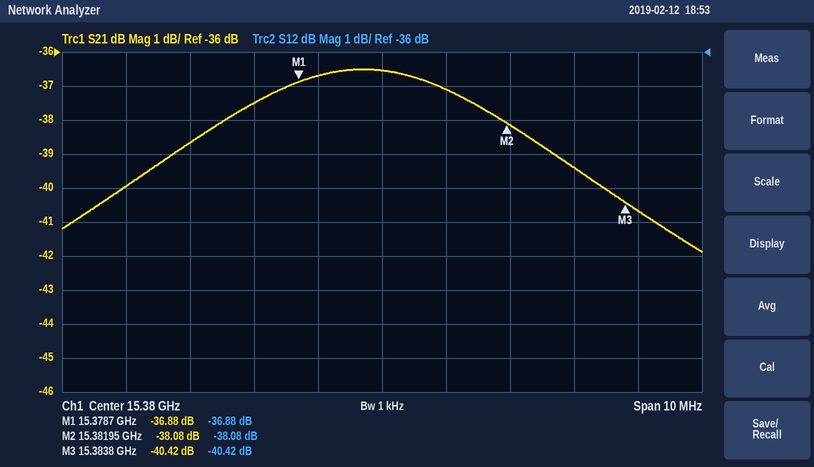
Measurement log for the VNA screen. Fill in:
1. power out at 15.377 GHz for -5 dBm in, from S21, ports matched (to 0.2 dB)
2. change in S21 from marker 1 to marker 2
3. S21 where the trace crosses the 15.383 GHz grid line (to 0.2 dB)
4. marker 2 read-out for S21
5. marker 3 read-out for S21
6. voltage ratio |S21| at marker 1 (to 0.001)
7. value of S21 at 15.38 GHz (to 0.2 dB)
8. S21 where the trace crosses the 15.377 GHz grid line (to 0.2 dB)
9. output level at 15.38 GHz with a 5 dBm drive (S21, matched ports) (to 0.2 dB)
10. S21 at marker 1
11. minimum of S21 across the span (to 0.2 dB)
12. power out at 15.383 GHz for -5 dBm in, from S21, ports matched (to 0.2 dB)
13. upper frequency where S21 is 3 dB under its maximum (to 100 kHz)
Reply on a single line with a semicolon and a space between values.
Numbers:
-43.6 dBm; -1.20 dB; -39.4 dB; -38.08 dB; -40.42 dB; 0.014; -36.6 dB; -38.6 dB; -31.6 dBm; -36.88 dB; -41.8 dB; -44.4 dBm; 15.3831 GHz
